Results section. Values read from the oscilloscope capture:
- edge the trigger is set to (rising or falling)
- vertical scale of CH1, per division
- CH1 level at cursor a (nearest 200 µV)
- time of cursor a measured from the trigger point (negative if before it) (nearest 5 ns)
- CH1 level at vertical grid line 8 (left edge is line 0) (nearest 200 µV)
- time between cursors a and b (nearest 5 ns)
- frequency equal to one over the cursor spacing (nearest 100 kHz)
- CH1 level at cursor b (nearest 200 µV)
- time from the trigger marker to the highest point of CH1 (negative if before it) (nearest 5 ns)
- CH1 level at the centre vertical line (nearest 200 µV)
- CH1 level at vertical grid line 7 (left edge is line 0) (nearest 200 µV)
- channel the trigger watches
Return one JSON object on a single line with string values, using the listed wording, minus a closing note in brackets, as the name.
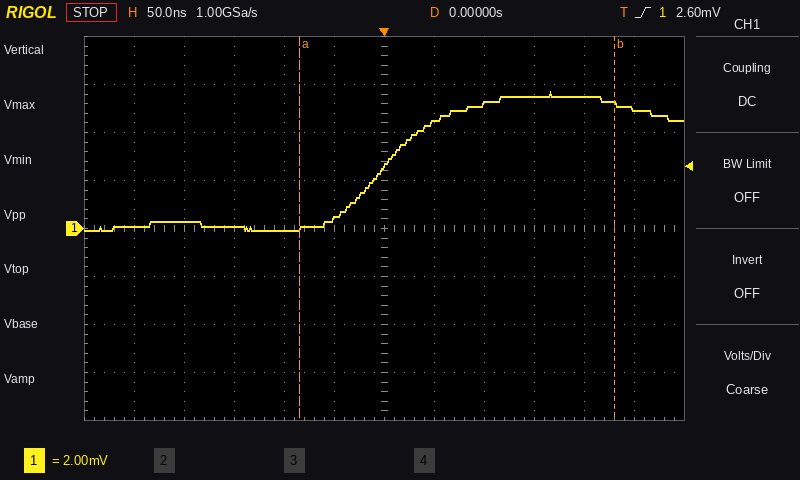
{"edge the trigger is set to": "rising", "vertical scale of CH1, per division": "2 mV", "CH1 level at cursor a": "0.0 mV", "time of cursor a measured from the trigger point (negative if before it)": "-85 ns", "CH1 level at vertical grid line 8 (left edge is line 0)": "5.2 mV", "time between cursors a and b": "315 ns", "frequency equal to one over the cursor spacing": "3.2 MHz", "CH1 level at cursor b": "5.2 mV", "time from the trigger marker to the highest point of CH1 (negative if before it)": "+165 ns", "CH1 level at the centre vertical line": "2.6 mV", "CH1 level at vertical grid line 7 (left edge is line 0)": "4.4 mV", "channel the trigger watches": "CH1"}
